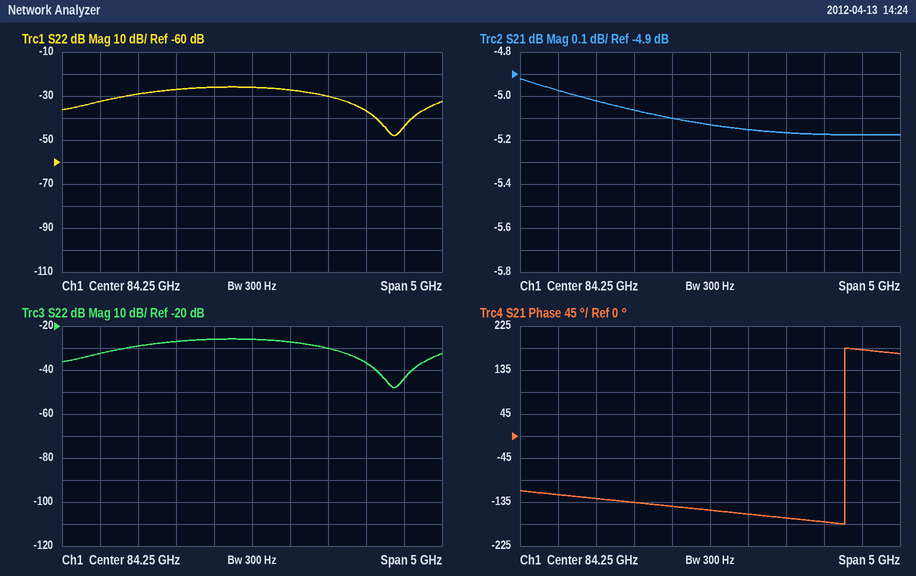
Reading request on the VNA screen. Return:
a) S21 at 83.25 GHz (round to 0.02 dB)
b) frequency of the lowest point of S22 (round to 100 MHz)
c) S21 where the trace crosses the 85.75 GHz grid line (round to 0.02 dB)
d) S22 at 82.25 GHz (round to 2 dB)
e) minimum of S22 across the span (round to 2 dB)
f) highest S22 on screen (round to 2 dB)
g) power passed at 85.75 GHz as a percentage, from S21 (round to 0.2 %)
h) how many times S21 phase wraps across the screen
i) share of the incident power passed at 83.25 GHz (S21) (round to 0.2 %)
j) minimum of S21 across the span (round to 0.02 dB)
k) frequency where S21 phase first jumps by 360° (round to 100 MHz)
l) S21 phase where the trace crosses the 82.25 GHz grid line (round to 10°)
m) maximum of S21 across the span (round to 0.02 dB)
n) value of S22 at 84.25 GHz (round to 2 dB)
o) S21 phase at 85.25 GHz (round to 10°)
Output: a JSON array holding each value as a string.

["-5.06 dB", "86.1 GHz", "-5.18 dB", "-32 dB", "-48 dB", "-26 dB", "30.4 %", "1", "31.2 %", "-5.18 dB", "86.0 GHz", "-120°", "-4.92 dB", "-26 dB", "-170°"]
